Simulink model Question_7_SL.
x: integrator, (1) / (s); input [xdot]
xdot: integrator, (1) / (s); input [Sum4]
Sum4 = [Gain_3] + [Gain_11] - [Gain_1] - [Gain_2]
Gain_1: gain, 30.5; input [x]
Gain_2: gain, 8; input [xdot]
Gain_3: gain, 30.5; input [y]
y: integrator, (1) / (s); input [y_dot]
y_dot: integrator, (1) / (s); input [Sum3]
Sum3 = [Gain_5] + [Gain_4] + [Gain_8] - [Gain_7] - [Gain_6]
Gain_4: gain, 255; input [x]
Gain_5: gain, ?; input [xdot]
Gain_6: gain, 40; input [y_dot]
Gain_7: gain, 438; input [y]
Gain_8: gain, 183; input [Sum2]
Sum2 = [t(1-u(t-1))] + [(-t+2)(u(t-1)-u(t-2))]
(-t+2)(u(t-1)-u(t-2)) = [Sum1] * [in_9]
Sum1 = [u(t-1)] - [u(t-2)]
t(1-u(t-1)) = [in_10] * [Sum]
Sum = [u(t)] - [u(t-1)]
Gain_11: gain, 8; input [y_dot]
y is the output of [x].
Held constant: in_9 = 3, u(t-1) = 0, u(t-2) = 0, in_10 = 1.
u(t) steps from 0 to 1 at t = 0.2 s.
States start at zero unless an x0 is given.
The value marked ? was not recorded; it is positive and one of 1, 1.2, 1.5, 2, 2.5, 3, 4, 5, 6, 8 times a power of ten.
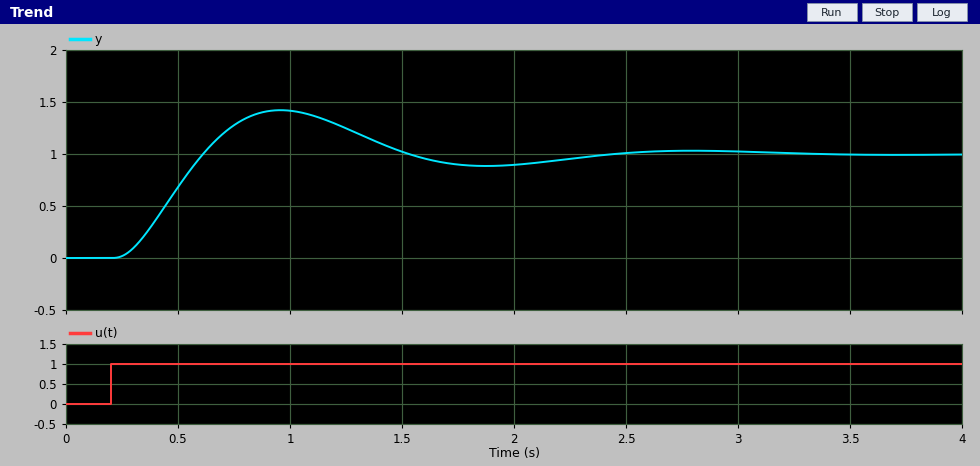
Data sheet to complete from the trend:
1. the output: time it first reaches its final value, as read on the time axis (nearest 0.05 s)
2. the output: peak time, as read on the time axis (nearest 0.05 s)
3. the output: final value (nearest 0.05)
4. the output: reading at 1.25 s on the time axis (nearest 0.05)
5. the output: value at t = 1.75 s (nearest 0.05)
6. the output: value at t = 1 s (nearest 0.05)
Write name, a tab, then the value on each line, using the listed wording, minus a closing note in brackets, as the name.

the output: time it first reaches its final value, as read on the time axis	0.60 s
the output: peak time, as read on the time axis	0.95 s
the output: final value	1.00
the output: reading at 1.25 s on the time axis	1.25
the output: value at t = 1.75 s	0.90
the output: value at t = 1 s	1.40
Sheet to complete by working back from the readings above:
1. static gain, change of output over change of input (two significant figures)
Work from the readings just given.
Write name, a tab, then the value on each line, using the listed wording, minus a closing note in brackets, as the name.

static gain, change of output over change of input	1.0
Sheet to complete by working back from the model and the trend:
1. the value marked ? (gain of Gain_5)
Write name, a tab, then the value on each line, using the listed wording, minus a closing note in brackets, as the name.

the value marked ?	30
